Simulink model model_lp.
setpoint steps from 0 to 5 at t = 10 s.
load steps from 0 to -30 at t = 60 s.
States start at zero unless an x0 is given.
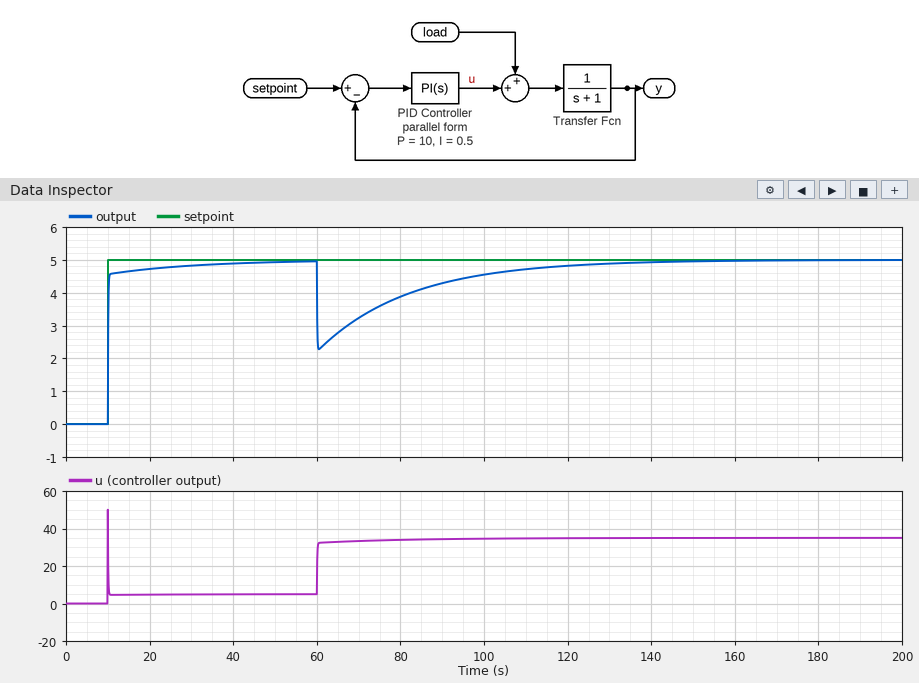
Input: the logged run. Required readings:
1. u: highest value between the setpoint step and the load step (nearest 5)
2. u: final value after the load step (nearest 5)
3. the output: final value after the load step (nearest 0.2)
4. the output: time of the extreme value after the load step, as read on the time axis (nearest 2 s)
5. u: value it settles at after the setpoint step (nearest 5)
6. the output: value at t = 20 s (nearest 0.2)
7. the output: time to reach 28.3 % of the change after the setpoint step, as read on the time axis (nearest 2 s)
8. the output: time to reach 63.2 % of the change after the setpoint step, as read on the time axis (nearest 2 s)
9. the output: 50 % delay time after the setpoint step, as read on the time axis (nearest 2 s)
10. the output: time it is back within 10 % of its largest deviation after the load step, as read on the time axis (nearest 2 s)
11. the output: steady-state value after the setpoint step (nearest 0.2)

50
35
5.0
60 s
5
4.8
10 s
10 s
10 s
112 s
5.0
